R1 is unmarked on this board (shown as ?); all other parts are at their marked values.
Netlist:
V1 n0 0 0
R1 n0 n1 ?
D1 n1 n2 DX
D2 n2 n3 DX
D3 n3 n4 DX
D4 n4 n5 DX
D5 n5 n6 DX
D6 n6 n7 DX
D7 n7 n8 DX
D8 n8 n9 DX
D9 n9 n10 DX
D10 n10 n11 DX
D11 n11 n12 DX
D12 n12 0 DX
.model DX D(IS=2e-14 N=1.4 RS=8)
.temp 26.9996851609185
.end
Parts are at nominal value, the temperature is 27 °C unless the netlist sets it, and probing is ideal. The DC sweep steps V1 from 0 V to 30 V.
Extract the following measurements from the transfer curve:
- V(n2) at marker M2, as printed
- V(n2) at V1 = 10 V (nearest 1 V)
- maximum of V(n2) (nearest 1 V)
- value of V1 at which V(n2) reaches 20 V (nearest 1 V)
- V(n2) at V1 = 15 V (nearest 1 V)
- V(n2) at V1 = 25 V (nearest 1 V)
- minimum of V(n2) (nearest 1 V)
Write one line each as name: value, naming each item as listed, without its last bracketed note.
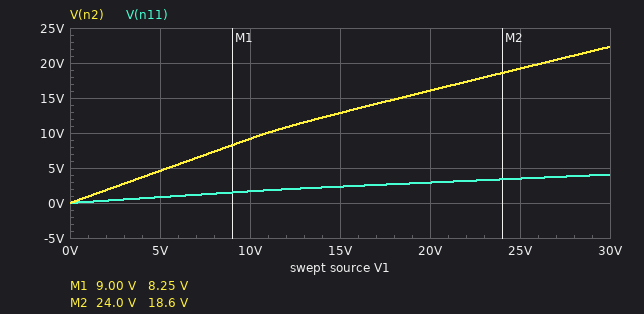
V(n2) at marker M2, as printed: 18.6 V
V(n2) at V1 = 10 V: 9 V
maximum of V(n2): 22 V
value of V1 at which V(n2) reaches 20 V: 26 V
V(n2) at V1 = 15 V: 13 V
V(n2) at V1 = 25 V: 19 V
minimum of V(n2): 0 V
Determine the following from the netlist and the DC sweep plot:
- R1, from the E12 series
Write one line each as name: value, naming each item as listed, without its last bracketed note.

R1, from the E12 series: 47 Ω
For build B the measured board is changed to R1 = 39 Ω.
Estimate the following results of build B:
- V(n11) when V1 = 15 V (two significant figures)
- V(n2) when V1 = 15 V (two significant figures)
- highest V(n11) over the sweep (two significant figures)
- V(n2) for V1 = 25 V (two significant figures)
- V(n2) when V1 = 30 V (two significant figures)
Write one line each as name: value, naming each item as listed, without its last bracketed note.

V(n11) when V1 = 15 V: 2.4 V
V(n2) when V1 = 15 V: 13 V
highest V(n11) over the sweep: 4.2 V
V(n2) for V1 = 25 V: 20 V
V(n2) when V1 = 30 V: 23 V
